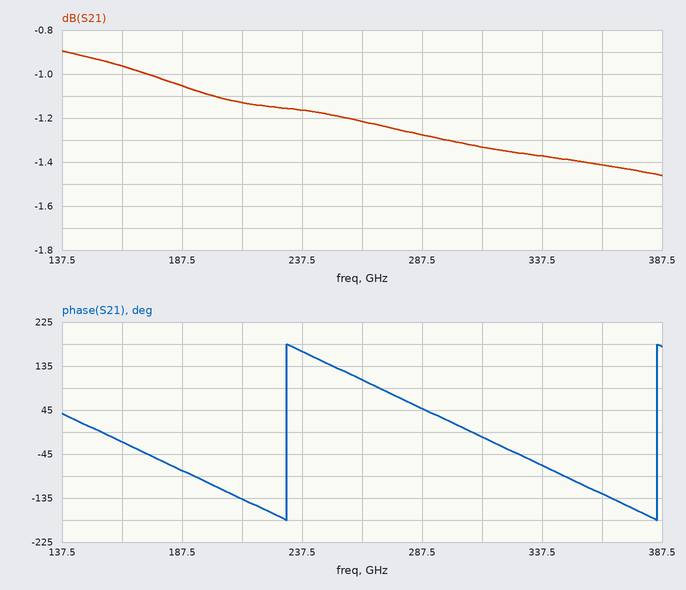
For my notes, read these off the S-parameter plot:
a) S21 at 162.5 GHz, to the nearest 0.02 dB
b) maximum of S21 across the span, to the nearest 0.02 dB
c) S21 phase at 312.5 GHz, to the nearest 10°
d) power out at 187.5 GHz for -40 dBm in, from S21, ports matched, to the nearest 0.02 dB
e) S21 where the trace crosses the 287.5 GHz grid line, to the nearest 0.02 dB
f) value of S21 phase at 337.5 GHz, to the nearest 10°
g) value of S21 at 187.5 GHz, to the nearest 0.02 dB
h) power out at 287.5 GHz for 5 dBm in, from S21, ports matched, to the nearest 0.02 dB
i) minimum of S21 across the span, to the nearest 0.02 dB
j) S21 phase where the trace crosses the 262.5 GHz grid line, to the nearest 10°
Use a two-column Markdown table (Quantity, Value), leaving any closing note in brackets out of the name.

| Quantity | Value |
|---|---|
| S21 at 162.5 GHz, to the nearest 0.02 dB | -0.96 dB |
| maximum of S21 across the span, to the nearest 0.02 dB | -0.90 dB |
| S21 phase at 312.5 GHz, to the nearest 10° | -10° |
| power out at 187.5 GHz for -40 dBm in, from S21, ports matched, to the nearest 0.02 dB | -41.06 dBm |
| S21 where the trace crosses the 287.5 GHz grid line, to the nearest 0.02 dB | -1.28 dB |
| value of S21 phase at 337.5 GHz, to the nearest 10° | -70° |
| value of S21 at 187.5 GHz, to the nearest 0.02 dB | -1.06 dB |
| power out at 287.5 GHz for 5 dBm in, from S21, ports matched, to the nearest 0.02 dB | 3.72 dBm |
| minimum of S21 across the span, to the nearest 0.02 dB | -1.46 dB |
| S21 phase where the trace crosses the 262.5 GHz grid line, to the nearest 10° | 110° |
